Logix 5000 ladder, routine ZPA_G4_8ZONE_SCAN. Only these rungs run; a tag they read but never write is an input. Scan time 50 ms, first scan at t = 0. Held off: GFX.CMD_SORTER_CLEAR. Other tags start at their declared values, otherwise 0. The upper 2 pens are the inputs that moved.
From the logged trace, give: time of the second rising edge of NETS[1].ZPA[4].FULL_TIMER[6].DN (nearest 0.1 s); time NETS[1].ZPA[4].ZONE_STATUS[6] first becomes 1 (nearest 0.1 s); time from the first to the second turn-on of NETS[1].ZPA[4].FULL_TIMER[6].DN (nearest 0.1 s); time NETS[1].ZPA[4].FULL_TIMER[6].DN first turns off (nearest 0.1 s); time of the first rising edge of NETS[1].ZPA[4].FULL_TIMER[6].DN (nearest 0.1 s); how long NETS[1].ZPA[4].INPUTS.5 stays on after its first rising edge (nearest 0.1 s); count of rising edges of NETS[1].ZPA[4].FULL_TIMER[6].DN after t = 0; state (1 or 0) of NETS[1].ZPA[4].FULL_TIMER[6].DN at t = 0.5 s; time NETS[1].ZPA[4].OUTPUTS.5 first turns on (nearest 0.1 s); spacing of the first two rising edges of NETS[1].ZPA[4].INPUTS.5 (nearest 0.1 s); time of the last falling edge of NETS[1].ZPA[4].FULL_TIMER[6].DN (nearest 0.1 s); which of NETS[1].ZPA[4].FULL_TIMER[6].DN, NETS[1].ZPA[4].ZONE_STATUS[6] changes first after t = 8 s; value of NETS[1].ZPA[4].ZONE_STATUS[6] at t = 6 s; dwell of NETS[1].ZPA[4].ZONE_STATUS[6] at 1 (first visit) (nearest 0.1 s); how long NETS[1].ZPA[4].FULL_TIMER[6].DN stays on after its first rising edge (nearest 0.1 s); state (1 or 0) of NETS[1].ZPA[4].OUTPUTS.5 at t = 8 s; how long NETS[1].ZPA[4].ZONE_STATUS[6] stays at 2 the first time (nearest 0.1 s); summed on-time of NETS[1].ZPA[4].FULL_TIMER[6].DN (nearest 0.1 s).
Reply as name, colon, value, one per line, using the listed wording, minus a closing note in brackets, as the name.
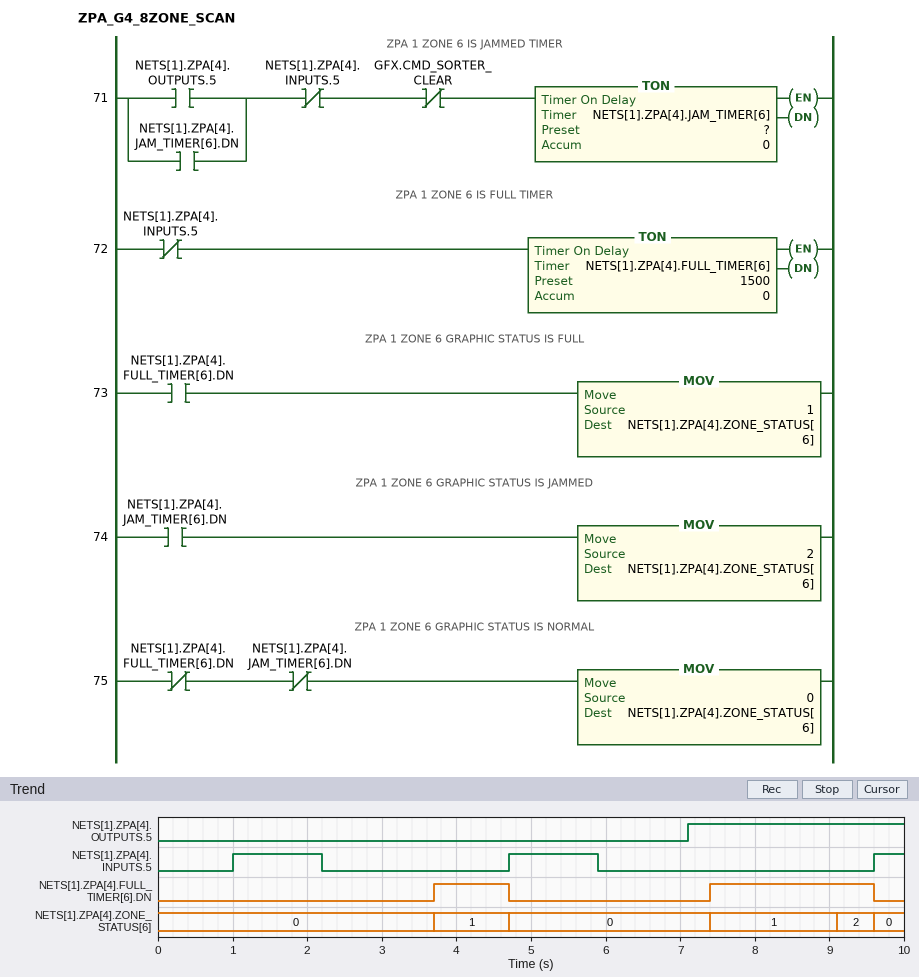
time of the second rising edge of NETS[1].ZPA[4].FULL_TIMER[6].DN: 7.4 s
time NETS[1].ZPA[4].ZONE_STATUS[6] first becomes 1: 3.7 s
time from the first to the second turn-on of NETS[1].ZPA[4].FULL_TIMER[6].DN: 3.7 s
time NETS[1].ZPA[4].FULL_TIMER[6].DN first turns off: 4.7 s
time of the first rising edge of NETS[1].ZPA[4].FULL_TIMER[6].DN: 3.7 s
how long NETS[1].ZPA[4].INPUTS.5 stays on after its first rising edge: 1.2 s
count of rising edges of NETS[1].ZPA[4].FULL_TIMER[6].DN after t = 0: 2
state (1 or 0) of NETS[1].ZPA[4].FULL_TIMER[6].DN at t = 0.5 s: 0
time NETS[1].ZPA[4].OUTPUTS.5 first turns on: 7.1 s
spacing of the first two rising edges of NETS[1].ZPA[4].INPUTS.5: 3.7 s
time of the last falling edge of NETS[1].ZPA[4].FULL_TIMER[6].DN: 9.6 s
which of NETS[1].ZPA[4].FULL_TIMER[6].DN, NETS[1].ZPA[4].ZONE_STATUS[6] changes first after t = 8 s: NETS[1].ZPA[4].ZONE_STATUS[6]
value of NETS[1].ZPA[4].ZONE_STATUS[6] at t = 6 s: 0
dwell of NETS[1].ZPA[4].ZONE_STATUS[6] at 1 (first visit): 1.0 s
how long NETS[1].ZPA[4].FULL_TIMER[6].DN stays on after its first rising edge: 1.0 s
state (1 or 0) of NETS[1].ZPA[4].OUTPUTS.5 at t = 8 s: 1
how long NETS[1].ZPA[4].ZONE_STATUS[6] stays at 2 the first time: 0.5 s
summed on-time of NETS[1].ZPA[4].FULL_TIMER[6].DN: 3.2 s
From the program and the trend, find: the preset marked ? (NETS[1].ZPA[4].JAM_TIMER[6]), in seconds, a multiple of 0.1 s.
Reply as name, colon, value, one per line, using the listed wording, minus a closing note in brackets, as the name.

the preset marked ? (NETS[1].ZPA[4].JAM_TIMER[6]), in seconds, a multiple of 0.1 s: 2.0 s
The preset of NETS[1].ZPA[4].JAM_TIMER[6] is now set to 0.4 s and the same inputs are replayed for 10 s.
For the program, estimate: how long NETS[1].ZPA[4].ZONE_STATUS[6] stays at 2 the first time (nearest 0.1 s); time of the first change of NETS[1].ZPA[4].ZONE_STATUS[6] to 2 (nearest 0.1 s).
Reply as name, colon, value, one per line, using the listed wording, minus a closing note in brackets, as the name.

how long NETS[1].ZPA[4].ZONE_STATUS[6] stays at 2 the first time: 2.1 s
time of the first change of NETS[1].ZPA[4].ZONE_STATUS[6] to 2: 7.5 s
